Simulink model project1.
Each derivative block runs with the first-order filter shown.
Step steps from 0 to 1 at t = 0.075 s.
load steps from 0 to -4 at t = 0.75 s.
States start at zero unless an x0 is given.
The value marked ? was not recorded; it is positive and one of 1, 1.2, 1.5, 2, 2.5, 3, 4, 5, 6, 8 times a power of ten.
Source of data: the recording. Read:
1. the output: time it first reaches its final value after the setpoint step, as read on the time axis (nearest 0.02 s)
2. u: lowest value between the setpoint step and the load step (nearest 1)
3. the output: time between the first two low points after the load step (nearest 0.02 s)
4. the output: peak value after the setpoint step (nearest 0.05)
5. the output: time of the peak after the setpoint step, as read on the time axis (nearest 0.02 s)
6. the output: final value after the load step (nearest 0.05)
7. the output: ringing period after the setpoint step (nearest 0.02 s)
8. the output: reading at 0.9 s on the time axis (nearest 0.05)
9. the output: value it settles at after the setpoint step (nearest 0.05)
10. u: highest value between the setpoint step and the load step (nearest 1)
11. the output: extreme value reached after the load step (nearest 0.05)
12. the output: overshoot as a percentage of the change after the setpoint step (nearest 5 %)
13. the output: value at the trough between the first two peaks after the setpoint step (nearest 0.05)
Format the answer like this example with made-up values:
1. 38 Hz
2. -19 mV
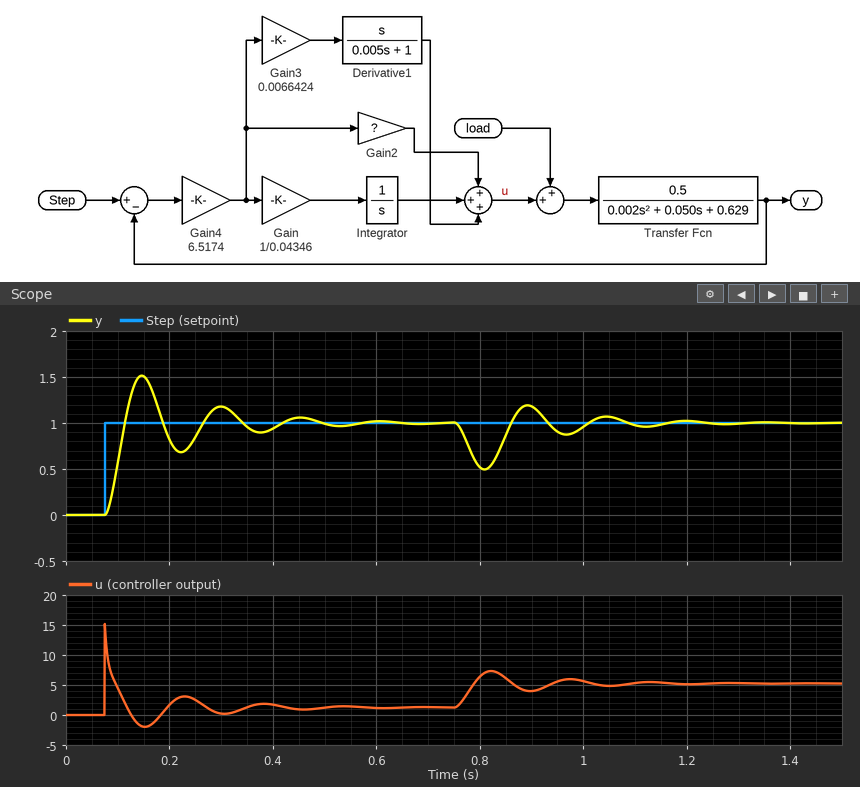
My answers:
1. 0.12 s
2. -2
3. 0.16 s
4. 1.50
5. 0.14 s
6. 1.00
7. 0.16 s
8. 1.20
9. 1.00
10. 15
11. 0.50
12. 50 %
13. 0.70
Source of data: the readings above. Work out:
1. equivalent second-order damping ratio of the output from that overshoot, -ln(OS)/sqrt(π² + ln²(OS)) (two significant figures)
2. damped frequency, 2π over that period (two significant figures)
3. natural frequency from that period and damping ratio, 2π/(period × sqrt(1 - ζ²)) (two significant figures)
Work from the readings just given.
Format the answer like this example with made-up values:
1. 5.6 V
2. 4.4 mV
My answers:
1. 0.22
2. 39 rad/s
3. 40 rad/s
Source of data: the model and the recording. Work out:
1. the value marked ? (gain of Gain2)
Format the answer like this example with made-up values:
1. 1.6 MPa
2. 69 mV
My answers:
1. 1
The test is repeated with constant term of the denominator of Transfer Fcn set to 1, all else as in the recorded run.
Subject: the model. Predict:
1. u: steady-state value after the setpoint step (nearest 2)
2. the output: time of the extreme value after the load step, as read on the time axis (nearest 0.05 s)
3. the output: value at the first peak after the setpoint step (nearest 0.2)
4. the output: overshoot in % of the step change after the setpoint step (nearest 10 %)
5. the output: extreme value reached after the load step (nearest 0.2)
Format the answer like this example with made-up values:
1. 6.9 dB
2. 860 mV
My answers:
1. 2
2. 0.80 s
3. 1.4
4. 40 %
5. 0.6
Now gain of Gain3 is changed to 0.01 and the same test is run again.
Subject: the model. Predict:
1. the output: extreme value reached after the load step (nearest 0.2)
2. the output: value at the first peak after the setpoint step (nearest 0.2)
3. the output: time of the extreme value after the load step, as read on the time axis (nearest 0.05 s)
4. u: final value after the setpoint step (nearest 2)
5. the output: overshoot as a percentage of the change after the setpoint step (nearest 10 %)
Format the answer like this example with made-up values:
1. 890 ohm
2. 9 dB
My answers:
1. 0.6
2. 1.4
3. 0.80 s
4. 2
5. 40 %
